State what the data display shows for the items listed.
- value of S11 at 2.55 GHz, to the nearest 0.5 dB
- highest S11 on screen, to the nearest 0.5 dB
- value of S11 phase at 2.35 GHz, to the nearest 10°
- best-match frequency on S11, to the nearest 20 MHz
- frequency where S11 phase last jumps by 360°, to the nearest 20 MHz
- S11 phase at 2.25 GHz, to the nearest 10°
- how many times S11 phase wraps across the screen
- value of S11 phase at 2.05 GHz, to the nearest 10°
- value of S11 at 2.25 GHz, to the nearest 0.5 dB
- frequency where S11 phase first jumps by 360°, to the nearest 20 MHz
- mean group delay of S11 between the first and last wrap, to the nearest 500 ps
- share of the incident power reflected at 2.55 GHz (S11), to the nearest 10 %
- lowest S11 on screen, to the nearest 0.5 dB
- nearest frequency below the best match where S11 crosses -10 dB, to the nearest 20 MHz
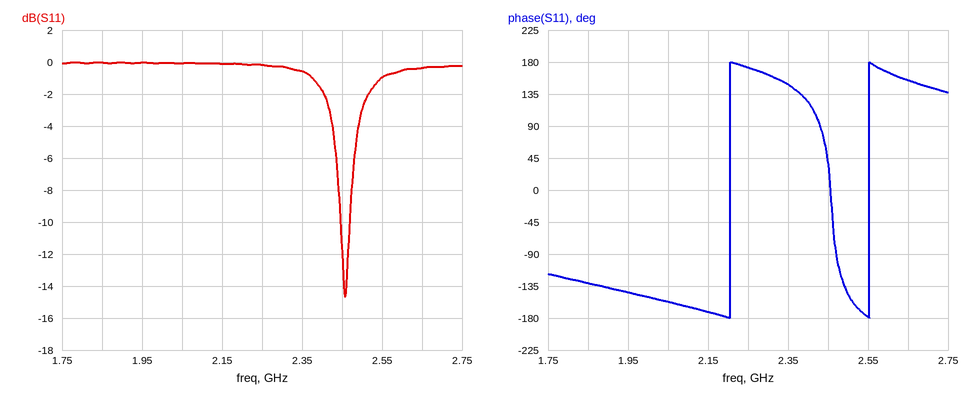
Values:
-1.0 dB
0.0 dB
150°
2.46 GHz
2.56 GHz
170°
2
-160°
0.0 dB
2.20 GHz
3.0 ns
80 %
-14.5 dB
2.44 GHz
